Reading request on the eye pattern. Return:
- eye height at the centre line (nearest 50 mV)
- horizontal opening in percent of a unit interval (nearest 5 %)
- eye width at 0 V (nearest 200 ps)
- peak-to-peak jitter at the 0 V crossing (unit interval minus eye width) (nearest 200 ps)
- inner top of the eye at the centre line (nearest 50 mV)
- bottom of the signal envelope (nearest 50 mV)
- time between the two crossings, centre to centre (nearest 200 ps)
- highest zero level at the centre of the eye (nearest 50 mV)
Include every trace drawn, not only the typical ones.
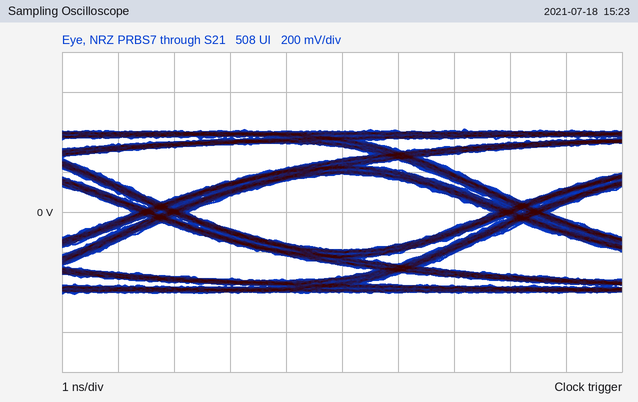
400 mV
85 %
5.4 ns
1.0 ns
200 mV
-400 mV
6.4 ns
-200 mV
